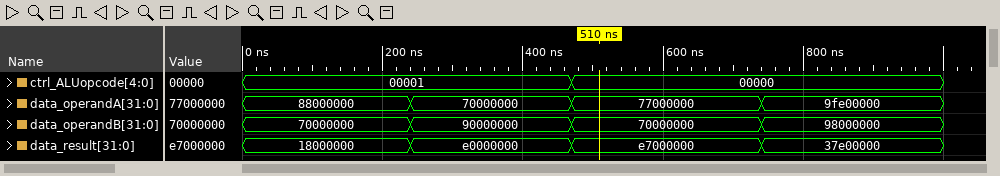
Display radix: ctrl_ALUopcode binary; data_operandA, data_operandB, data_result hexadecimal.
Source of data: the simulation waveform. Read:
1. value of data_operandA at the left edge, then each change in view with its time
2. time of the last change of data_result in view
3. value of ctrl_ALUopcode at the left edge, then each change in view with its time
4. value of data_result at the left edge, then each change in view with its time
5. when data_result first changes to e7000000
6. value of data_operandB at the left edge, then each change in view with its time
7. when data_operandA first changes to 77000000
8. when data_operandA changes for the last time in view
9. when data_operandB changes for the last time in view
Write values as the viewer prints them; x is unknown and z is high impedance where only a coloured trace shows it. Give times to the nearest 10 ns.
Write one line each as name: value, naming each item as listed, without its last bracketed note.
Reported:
value of data_operandA at the left edge, then each change in view with its time: 88000000, 70000000 at 240 ns, 77000000 at 470 ns, 9fe00000 at 740 ns
time of the last change of data_result in view: 740 ns
value of ctrl_ALUopcode at the left edge, then each change in view with its time: 00001, 00000 at 470 ns
value of data_result at the left edge, then each change in view with its time: 18000000, e0000000 at 240 ns, e7000000 at 470 ns, 37e00000 at 740 ns
when data_result first changes to e7000000: 470 ns
value of data_operandB at the left edge, then each change in view with its time: 70000000, 90000000 at 240 ns, 70000000 at 470 ns, 98000000 at 740 ns
when data_operandA first changes to 77000000: 470 ns
when data_operandA changes for the last time in view: 740 ns
when data_operandB changes for the last time in view: 740 ns
